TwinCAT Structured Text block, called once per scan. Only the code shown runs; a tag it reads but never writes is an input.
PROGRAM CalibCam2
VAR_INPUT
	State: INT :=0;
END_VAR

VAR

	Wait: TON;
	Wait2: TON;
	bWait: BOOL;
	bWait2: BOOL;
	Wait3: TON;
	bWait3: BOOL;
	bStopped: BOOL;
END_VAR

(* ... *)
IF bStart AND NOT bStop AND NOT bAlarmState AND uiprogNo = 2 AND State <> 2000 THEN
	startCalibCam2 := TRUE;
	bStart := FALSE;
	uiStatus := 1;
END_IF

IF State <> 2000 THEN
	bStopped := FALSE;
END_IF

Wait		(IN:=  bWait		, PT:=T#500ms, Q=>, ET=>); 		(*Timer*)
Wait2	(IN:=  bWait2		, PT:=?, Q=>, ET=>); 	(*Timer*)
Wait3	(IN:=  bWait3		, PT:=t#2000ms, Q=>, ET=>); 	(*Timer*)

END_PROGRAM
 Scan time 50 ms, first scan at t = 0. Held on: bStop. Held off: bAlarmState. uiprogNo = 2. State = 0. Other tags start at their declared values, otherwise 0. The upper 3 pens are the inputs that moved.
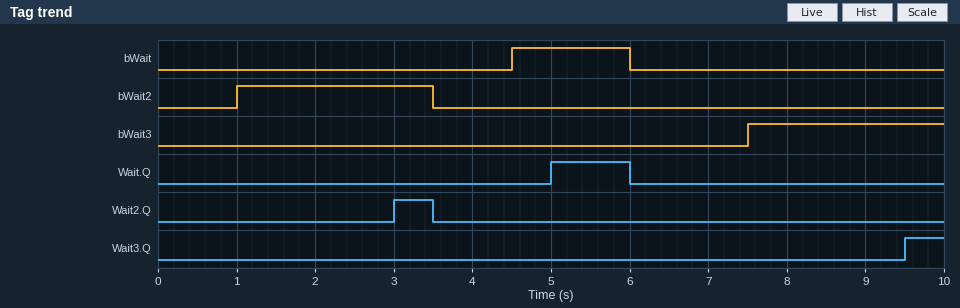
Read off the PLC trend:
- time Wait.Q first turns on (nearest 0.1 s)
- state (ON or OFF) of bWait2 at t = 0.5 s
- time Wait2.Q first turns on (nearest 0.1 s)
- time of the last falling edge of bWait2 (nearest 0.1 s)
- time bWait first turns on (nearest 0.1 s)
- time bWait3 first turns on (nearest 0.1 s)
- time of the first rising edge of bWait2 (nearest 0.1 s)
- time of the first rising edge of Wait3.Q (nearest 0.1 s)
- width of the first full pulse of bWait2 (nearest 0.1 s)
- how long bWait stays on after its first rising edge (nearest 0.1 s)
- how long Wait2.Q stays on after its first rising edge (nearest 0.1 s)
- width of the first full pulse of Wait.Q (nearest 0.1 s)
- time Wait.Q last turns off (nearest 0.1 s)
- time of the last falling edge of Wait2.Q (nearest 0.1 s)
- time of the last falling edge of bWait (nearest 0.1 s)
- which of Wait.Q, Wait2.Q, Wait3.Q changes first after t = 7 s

5.0 s
OFF
3.0 s
3.5 s
4.5 s
7.5 s
1.0 s
9.5 s
2.5 s
1.5 s
0.5 s
1.0 s
6.0 s
3.5 s
6.0 s
Wait3.Q
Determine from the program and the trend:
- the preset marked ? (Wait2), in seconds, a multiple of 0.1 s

2.0 s
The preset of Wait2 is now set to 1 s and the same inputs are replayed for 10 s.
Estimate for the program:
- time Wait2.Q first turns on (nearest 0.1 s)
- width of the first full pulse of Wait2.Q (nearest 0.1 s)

2.0 s
1.5 s
